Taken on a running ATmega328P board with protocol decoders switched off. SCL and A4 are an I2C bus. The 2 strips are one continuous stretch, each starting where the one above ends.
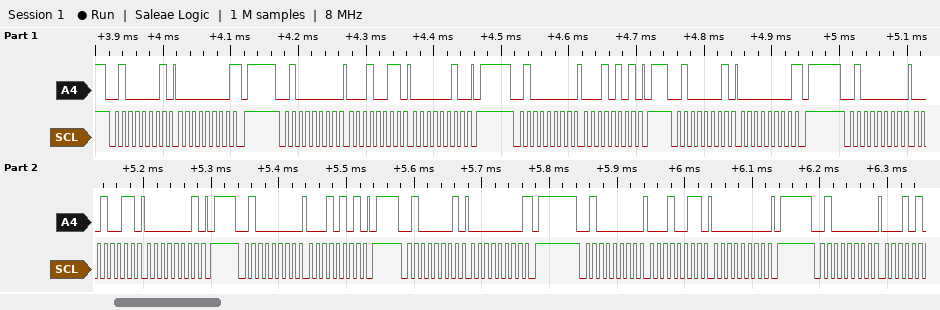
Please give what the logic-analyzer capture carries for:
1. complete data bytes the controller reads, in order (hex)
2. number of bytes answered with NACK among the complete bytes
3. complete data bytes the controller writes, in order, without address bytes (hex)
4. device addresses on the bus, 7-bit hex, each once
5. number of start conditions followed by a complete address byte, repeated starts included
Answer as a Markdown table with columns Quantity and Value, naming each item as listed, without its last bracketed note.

| Quantity | Value |
|---|---|
| complete data bytes the controller reads, in order | 00 00 00 |
| number of bytes answered with NACK among the complete bytes | 3 |
| complete data bytes the controller writes, in order, without address bytes | 13 02 15 13 01 15 13 00 |
| device addresses on the bus, 7-bit hex, each once | 0x20 |
| number of start conditions followed by a complete address byte, repeated starts included | 9 |
